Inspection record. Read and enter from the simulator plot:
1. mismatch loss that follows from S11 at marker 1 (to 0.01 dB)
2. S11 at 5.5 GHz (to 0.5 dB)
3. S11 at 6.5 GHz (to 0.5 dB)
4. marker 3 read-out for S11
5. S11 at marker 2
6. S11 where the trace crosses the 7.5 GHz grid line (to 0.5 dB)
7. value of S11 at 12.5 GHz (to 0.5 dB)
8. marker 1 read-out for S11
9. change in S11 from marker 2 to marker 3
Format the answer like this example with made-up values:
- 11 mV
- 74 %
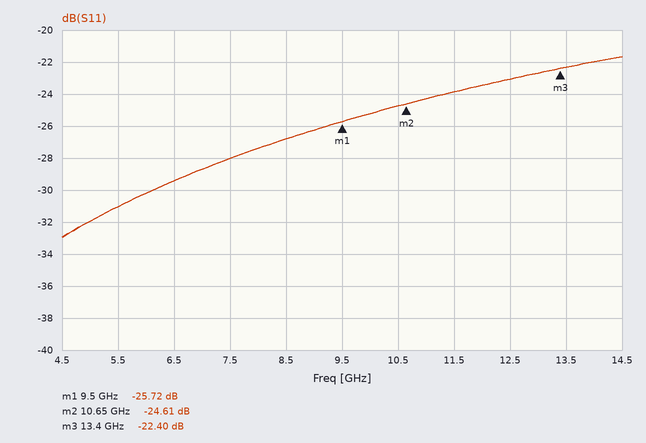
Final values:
- 0.01 dB
- -31.0 dB
- -29.5 dB
- -22.40 dB
- -24.61 dB
- -28.0 dB
- -23.0 dB
- -25.72 dB
- 2.21 dB
